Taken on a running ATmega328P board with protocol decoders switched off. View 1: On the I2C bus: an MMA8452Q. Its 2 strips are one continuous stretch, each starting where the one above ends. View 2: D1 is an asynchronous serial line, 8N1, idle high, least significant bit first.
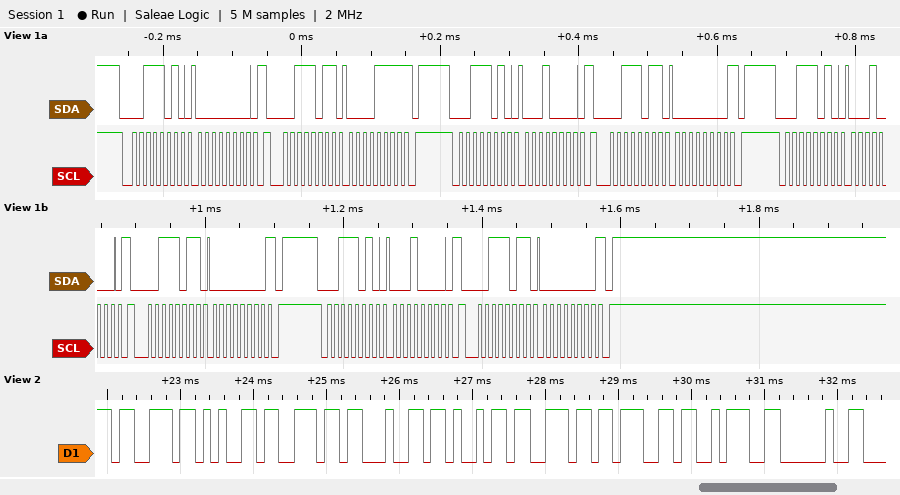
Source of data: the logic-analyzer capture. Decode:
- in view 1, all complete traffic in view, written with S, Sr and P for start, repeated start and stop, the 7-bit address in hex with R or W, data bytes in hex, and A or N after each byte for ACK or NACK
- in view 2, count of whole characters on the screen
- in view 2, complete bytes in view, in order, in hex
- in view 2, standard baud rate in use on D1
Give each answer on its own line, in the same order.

S 1DW A 00 A Sr 1DR A 0F N P S 1DW A 10 A Sr 1DR A 00 N P S 1DW A 10 A Sr 1DR A 00 N P S 1DW A 10 A Sr 1DR A 00 N P
9
73 65 6E 64 69 6E 67 3A 20
9600 baud
